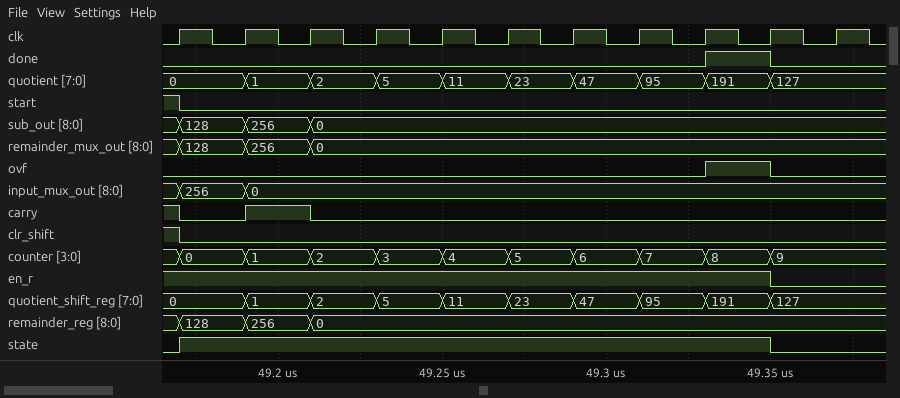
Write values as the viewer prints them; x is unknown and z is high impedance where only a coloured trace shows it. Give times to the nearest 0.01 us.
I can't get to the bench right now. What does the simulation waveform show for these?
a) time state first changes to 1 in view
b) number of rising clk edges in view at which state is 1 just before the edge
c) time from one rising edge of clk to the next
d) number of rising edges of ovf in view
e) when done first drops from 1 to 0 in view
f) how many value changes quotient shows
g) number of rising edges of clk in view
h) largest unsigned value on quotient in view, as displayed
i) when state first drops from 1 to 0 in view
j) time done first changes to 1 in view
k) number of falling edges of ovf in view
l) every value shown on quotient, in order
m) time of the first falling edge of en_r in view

49.17 us
9
0.02 us
1
49.35 us
9
11
191
49.35 us
49.33 us
1
0, 1, 2, 5, 11, 23, 47, 95, 191, 127
49.35 us
